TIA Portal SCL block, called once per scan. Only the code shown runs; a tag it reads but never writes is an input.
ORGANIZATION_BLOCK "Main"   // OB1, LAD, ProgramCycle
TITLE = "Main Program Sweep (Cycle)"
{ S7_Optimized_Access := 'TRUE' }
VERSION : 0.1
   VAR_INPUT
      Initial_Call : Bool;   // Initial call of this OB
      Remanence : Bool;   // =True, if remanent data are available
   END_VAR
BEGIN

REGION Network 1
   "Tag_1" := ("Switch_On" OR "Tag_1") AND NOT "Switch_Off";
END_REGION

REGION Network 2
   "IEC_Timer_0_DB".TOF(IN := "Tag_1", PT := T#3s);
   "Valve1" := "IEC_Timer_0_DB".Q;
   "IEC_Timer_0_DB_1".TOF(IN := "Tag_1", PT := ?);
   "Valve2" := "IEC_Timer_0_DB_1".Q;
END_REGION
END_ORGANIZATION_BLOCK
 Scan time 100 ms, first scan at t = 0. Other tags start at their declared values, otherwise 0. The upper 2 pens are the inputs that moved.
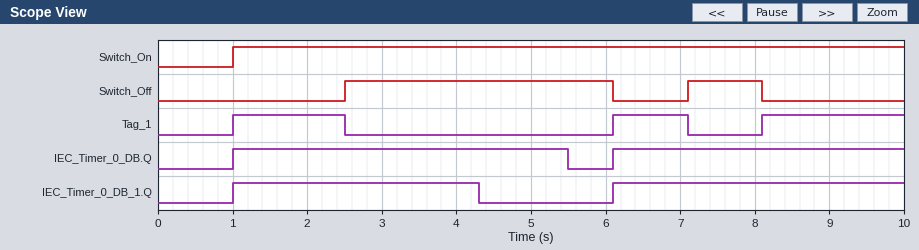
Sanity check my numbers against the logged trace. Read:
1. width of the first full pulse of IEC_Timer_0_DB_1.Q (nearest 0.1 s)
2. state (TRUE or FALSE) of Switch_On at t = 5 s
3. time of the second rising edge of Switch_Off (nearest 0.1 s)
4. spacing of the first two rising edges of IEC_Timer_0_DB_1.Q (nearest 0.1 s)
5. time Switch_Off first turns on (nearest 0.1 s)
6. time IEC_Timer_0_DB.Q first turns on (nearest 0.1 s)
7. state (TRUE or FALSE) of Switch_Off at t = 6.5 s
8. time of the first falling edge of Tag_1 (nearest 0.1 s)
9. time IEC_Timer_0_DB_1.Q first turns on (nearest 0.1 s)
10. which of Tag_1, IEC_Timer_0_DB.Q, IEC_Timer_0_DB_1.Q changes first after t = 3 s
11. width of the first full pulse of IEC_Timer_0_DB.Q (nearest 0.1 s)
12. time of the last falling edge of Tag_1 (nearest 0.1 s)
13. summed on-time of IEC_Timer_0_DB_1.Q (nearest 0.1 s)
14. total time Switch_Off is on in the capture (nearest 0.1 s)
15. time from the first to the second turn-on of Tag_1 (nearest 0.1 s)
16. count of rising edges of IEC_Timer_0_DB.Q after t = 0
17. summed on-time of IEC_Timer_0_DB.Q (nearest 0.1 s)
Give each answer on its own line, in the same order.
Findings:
3.3 s
TRUE
7.1 s
5.1 s
2.5 s
1.0 s
FALSE
2.5 s
1.0 s
IEC_Timer_0_DB_1.Q
4.5 s
7.1 s
7.2 s
4.6 s
5.1 s
2
8.4 s
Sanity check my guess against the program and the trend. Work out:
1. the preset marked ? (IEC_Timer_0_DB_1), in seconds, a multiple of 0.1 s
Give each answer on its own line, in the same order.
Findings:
1.8 s
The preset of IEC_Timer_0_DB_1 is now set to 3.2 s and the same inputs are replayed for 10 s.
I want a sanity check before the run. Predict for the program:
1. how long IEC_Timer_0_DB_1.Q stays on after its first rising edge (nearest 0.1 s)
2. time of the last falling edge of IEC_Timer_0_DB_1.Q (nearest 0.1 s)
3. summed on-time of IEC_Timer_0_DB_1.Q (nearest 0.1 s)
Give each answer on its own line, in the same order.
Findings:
4.7 s
5.7 s
8.6 s
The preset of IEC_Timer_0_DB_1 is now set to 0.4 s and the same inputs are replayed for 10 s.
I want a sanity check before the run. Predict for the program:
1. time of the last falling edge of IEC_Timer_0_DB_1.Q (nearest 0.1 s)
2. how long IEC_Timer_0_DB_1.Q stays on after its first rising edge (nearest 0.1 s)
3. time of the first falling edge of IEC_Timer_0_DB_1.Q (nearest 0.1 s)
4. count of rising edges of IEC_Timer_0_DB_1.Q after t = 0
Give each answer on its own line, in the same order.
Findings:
7.5 s
1.9 s
2.9 s
3
